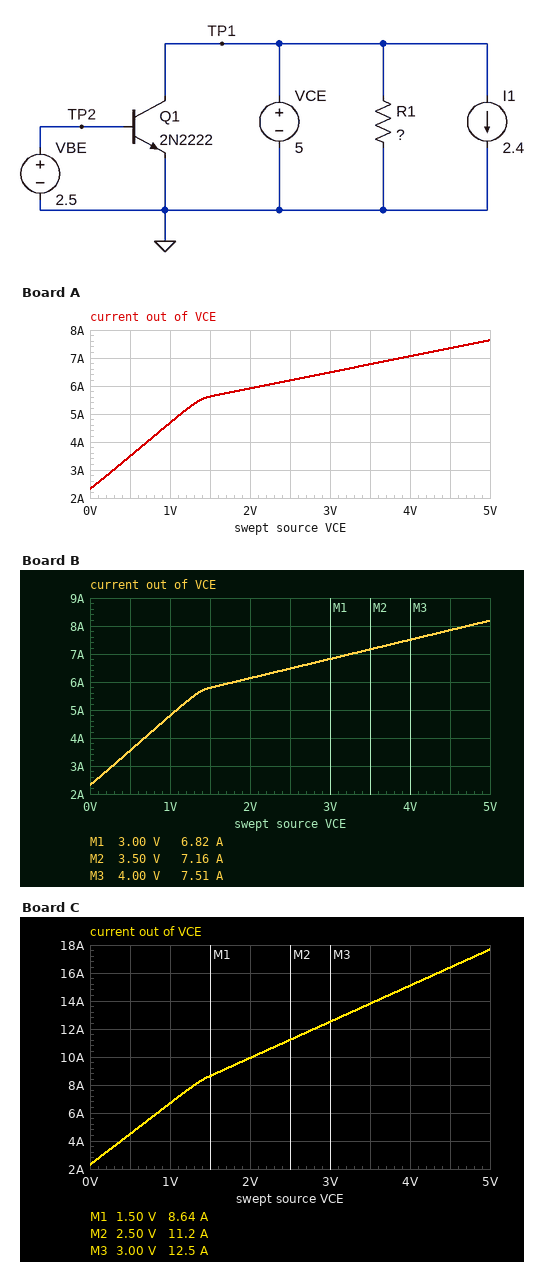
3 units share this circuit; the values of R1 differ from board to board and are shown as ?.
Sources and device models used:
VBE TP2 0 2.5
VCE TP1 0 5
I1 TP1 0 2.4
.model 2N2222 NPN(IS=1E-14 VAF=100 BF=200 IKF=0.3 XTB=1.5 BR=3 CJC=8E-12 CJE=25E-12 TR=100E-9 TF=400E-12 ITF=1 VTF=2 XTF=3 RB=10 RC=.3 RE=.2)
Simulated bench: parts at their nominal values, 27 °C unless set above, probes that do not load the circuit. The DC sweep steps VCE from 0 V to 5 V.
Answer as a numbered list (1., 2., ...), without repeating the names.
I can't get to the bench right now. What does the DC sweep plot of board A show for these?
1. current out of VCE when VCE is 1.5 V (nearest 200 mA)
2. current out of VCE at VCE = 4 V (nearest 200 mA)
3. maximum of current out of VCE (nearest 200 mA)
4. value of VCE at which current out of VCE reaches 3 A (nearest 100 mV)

1. 5.6 A
2. 7.0 A
3. 7.6 A
4. 300 mV
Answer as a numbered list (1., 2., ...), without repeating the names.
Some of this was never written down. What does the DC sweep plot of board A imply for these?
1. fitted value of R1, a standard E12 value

1. 1.8 Ω
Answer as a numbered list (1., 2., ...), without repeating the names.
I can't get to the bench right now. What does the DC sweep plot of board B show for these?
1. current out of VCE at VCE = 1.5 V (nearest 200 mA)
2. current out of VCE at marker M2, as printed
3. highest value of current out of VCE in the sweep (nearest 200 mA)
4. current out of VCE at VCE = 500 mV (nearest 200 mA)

1. 5.8 A
2. 7.16 A
3. 8.2 A
4. 3.6 A
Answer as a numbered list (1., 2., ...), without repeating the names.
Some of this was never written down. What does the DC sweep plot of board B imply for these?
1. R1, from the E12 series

1. 1.5 Ω
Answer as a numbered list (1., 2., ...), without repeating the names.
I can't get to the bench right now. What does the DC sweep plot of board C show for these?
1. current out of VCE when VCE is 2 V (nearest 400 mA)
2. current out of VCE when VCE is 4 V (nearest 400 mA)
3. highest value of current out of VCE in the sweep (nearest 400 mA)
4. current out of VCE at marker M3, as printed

1. 10.0 A
2. 15.2 A
3. 17.6 A
4. 12.5 A
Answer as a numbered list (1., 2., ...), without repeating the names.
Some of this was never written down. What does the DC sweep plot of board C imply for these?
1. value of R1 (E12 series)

1. 0.39 Ω
